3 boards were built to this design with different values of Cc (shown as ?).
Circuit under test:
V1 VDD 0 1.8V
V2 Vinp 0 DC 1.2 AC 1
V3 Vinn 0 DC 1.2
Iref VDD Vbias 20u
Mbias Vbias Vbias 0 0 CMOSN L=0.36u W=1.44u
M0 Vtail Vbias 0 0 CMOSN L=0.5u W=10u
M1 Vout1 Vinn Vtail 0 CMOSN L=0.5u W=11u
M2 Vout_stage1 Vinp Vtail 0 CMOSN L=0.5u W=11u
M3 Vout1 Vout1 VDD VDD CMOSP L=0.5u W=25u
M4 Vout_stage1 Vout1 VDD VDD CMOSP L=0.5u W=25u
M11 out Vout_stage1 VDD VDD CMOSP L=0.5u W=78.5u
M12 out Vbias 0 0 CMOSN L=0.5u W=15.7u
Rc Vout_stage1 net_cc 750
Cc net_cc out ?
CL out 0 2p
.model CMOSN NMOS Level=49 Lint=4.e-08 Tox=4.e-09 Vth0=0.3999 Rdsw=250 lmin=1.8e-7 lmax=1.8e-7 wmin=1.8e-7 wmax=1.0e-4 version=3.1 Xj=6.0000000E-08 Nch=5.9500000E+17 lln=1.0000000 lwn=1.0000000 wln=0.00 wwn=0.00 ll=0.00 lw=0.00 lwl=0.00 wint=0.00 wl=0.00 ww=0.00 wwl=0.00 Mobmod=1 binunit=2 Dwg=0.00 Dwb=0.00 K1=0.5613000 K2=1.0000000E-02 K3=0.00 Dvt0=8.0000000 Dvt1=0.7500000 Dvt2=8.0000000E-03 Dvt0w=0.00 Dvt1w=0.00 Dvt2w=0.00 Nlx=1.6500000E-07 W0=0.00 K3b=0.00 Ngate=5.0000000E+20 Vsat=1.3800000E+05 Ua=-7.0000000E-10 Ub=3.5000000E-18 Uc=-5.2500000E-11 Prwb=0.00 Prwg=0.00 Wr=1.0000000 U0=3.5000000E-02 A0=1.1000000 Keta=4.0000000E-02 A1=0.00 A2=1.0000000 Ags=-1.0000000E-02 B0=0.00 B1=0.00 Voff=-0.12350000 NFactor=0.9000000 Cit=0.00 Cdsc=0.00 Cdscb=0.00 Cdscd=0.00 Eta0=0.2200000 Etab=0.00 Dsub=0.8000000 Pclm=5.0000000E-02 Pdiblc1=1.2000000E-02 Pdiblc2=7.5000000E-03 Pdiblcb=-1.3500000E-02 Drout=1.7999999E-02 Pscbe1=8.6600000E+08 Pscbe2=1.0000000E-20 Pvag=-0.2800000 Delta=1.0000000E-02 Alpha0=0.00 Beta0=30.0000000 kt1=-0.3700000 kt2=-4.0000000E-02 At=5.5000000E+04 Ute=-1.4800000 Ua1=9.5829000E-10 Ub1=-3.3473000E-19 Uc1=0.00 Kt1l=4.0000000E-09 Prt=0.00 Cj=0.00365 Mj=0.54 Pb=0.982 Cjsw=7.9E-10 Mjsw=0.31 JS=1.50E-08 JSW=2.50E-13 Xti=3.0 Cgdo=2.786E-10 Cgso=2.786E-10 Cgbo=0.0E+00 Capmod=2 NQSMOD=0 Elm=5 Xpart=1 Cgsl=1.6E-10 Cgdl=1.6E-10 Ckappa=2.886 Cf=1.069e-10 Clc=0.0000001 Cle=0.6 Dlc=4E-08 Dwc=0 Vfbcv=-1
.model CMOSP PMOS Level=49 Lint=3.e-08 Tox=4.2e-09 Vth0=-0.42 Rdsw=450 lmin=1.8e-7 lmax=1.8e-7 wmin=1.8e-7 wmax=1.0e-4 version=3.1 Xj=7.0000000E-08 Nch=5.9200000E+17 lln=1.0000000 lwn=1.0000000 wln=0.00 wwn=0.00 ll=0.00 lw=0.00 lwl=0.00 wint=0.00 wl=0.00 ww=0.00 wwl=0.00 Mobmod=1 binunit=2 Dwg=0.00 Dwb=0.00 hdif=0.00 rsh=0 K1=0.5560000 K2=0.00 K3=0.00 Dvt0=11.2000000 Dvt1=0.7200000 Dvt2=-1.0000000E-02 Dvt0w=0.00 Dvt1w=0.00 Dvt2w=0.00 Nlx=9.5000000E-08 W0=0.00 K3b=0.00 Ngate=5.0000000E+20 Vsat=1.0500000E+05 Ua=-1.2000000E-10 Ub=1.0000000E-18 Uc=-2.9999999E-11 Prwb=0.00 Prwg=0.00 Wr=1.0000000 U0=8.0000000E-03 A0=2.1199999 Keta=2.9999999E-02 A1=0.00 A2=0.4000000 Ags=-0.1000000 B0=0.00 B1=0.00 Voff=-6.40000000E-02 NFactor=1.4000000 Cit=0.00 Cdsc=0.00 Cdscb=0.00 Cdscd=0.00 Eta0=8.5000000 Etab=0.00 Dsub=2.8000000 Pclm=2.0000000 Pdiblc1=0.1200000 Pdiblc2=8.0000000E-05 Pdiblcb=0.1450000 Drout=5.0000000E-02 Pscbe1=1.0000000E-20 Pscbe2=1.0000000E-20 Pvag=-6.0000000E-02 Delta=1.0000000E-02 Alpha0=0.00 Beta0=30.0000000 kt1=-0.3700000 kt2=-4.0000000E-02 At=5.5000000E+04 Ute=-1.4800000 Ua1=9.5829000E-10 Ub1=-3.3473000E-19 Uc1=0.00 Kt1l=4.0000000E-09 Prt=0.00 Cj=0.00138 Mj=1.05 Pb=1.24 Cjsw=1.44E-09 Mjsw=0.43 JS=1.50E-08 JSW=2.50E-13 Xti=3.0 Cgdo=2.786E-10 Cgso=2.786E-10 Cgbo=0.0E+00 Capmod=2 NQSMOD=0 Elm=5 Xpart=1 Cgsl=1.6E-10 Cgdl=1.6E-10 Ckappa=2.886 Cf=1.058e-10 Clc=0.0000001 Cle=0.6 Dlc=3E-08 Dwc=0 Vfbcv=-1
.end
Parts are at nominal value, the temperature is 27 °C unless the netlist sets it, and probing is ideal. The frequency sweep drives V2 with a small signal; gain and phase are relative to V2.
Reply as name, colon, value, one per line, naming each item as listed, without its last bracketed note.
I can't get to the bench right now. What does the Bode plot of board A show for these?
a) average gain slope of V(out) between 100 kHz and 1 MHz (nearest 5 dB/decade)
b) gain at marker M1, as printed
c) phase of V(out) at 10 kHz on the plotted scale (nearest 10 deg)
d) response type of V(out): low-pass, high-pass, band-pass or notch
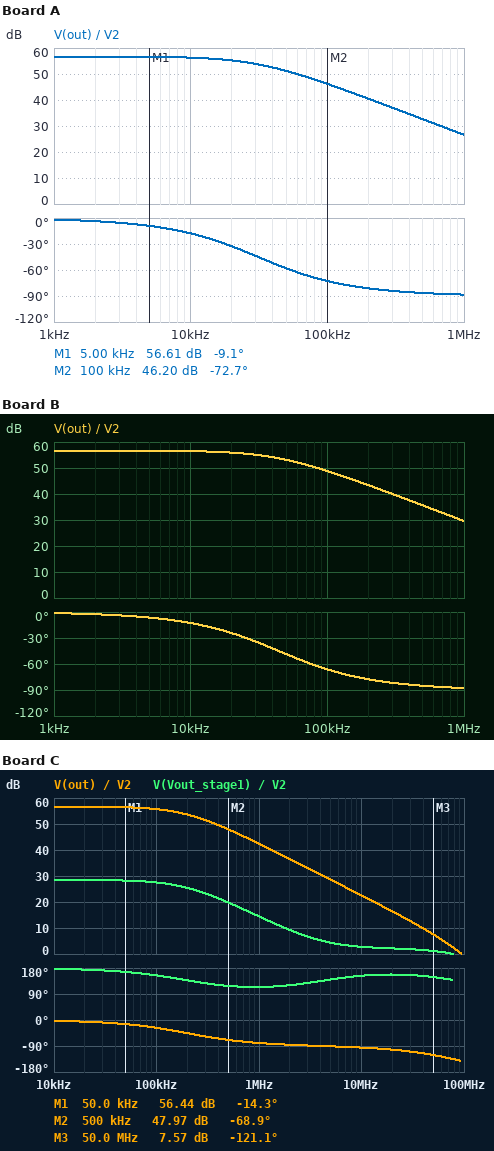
average gain slope of V(out) between 100 kHz and 1 MHz: -20 dB/decade
gain at marker M1, as printed: 56.61 dB
phase of V(out) at 10 kHz on the plotted scale: -20 deg
response type of V(out): low-pass, high-pass, band-pass or notch: low-pass
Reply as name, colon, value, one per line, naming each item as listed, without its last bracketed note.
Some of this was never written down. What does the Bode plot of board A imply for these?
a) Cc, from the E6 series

Cc, from the E6 series: 4.7 pF
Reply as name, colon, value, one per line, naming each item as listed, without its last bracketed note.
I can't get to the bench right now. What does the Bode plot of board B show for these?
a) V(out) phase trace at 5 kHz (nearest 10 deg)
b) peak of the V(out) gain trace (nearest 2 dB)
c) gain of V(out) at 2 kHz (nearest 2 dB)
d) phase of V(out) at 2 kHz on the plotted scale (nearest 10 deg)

V(out) phase trace at 5 kHz: -10 deg
peak of the V(out) gain trace: 56 dB
gain of V(out) at 2 kHz: 56 dB
phase of V(out) at 2 kHz on the plotted scale: 0 deg
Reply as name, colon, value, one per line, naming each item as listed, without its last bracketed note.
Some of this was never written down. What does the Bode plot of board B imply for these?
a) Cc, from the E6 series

Cc, from the E6 series: 3.3 pF
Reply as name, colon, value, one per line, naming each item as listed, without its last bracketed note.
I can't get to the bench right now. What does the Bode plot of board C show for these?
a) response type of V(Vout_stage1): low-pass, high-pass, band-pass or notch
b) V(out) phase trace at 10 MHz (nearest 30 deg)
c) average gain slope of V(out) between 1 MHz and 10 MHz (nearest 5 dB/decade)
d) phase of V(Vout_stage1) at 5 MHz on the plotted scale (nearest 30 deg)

response type of V(Vout_stage1): low-pass, high-pass, band-pass or notch: low-pass
V(out) phase trace at 10 MHz: -90 deg
average gain slope of V(out) between 1 MHz and 10 MHz: -20 dB/decade
phase of V(Vout_stage1) at 5 MHz on the plotted scale: 150 deg
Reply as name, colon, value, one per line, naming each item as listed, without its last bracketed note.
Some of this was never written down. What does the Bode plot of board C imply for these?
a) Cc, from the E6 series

Cc, from the E6 series: 680 fF
